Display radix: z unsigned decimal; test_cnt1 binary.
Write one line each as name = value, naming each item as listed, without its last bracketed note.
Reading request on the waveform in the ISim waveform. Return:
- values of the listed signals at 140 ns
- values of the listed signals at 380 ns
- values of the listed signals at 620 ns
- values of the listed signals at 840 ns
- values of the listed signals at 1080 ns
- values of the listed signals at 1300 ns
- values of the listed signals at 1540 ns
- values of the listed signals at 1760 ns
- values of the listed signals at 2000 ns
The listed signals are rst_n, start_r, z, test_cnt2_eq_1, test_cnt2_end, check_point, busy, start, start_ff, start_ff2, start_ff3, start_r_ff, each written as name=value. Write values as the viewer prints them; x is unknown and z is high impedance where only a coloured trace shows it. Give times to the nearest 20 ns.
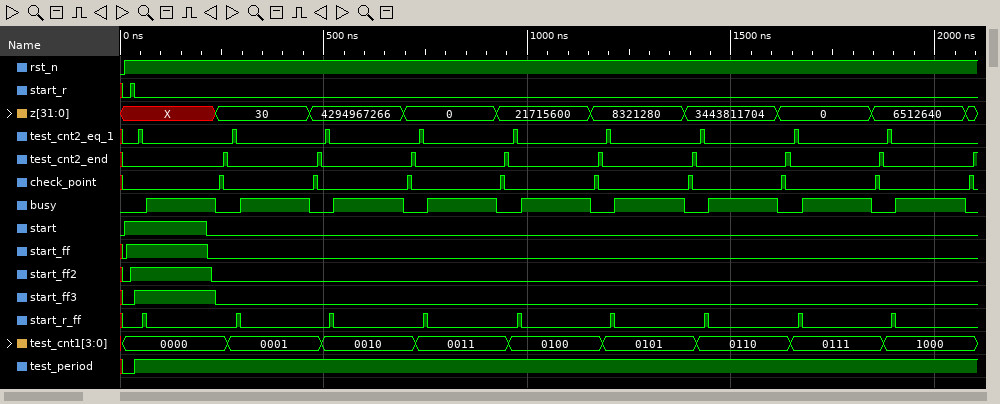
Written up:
values of the listed signals at 140 ns = rst_n=1, start_r=0, z=X, test_cnt2_eq_1=0, test_cnt2_end=0, check_point=0, busy=1, start=1, start_ff=1, start_ff2=1, start_ff3=1, start_r_ff=0
values of the listed signals at 380 ns = rst_n=1, start_r=0, z=30, test_cnt2_eq_1=0, test_cnt2_end=0, check_point=0, busy=1, start=0, start_ff=0, start_ff2=0, start_ff3=0, start_r_ff=0
values of the listed signals at 620 ns = rst_n=1, start_r=0, z=4294967266, test_cnt2_eq_1=0, test_cnt2_end=0, check_point=0, busy=1, start=0, start_ff=0, start_ff2=0, start_ff3=0, start_r_ff=0
values of the listed signals at 840 ns = rst_n=1, start_r=0, z=0, test_cnt2_eq_1=0, test_cnt2_end=0, check_point=0, busy=1, start=0, start_ff=0, start_ff2=0, start_ff3=0, start_r_ff=0
values of the listed signals at 1080 ns = rst_n=1, start_r=0, z=21715600, test_cnt2_eq_1=0, test_cnt2_end=0, check_point=0, busy=1, start=0, start_ff=0, start_ff2=0, start_ff3=0, start_r_ff=0
values of the listed signals at 1300 ns = rst_n=1, start_r=0, z=8321280, test_cnt2_eq_1=0, test_cnt2_end=0, check_point=0, busy=1, start=0, start_ff=0, start_ff2=0, start_ff3=0, start_r_ff=0
values of the listed signals at 1540 ns = rst_n=1, start_r=0, z=3443811704, test_cnt2_eq_1=0, test_cnt2_end=0, check_point=0, busy=1, start=0, start_ff=0, start_ff2=0, start_ff3=0, start_r_ff=0
values of the listed signals at 1760 ns = rst_n=1, start_r=0, z=0, test_cnt2_eq_1=0, test_cnt2_end=0, check_point=0, busy=1, start=0, start_ff=0, start_ff2=0, start_ff3=0, start_r_ff=0
values of the listed signals at 2000 ns = rst_n=1, start_r=0, z=6512640, test_cnt2_eq_1=0, test_cnt2_end=0, check_point=0, busy=1, start=0, start_ff=0, start_ff2=0, start_ff3=0, start_r_ff=0
